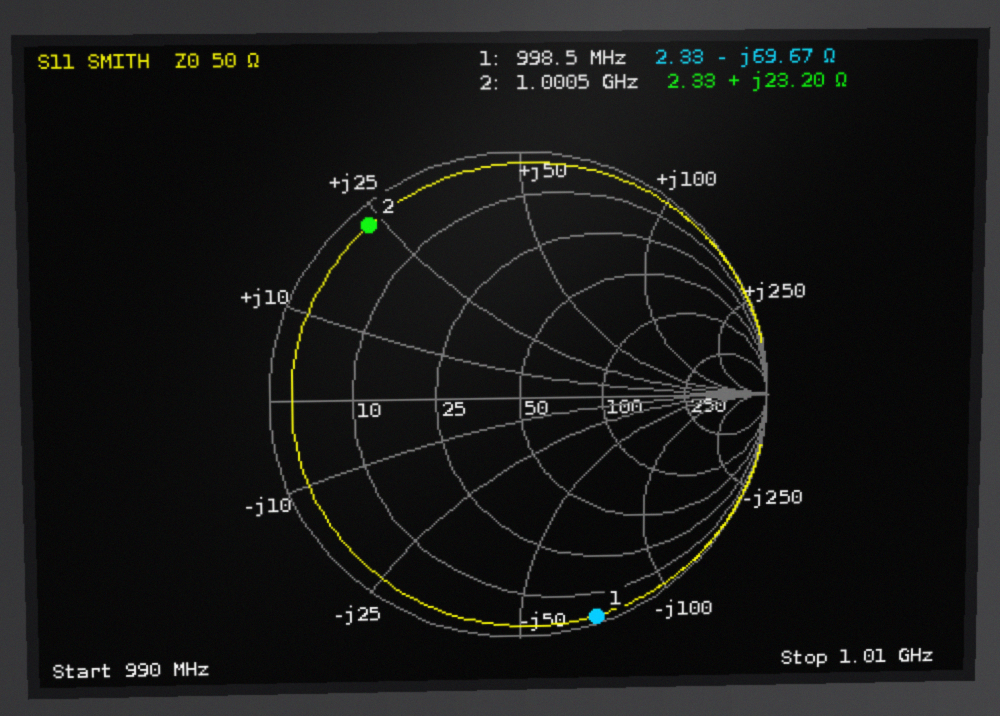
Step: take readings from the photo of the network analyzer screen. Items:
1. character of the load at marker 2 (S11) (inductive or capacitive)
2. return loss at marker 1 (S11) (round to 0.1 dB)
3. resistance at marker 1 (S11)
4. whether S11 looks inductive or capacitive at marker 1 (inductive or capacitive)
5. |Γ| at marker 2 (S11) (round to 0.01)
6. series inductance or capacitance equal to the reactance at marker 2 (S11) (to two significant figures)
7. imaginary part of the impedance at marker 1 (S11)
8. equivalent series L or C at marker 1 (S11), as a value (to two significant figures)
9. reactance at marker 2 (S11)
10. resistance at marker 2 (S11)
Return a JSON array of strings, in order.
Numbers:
["inductive", "0.3 dB", "2.33 Ω", "capacitive", "0.93", "3.7 nH", "-69.67 Ω", "2.3 pF", "+23.20 Ω", "2.33 Ω"]
